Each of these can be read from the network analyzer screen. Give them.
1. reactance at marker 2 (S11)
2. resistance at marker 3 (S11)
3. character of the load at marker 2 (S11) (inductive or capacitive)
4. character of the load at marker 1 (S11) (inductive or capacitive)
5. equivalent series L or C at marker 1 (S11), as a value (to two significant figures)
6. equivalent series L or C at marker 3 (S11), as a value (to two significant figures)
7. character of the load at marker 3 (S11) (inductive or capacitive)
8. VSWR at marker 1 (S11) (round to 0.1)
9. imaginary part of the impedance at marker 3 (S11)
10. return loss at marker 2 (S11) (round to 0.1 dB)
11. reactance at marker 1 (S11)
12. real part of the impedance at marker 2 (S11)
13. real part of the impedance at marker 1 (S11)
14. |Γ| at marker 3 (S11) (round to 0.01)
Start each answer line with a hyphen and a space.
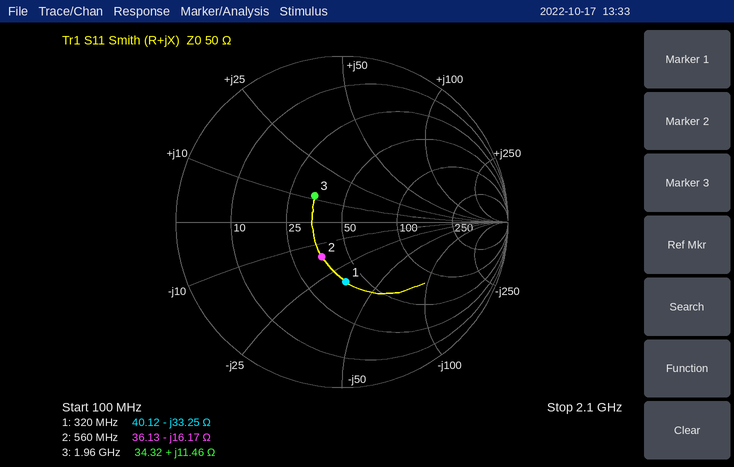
- -16.17 Ω
- 34.32 Ω
- capacitive
- capacitive
- 15 pF
- 930 pH
- inductive
- 2.1
- +11.46 Ω
- 12.3 dB
- -33.25 Ω
- 36.13 Ω
- 40.12 Ω
- 0.23
